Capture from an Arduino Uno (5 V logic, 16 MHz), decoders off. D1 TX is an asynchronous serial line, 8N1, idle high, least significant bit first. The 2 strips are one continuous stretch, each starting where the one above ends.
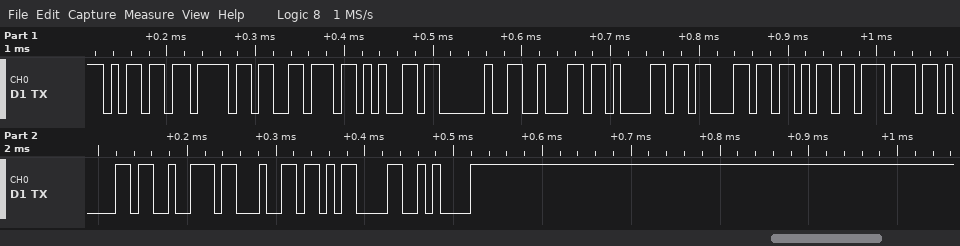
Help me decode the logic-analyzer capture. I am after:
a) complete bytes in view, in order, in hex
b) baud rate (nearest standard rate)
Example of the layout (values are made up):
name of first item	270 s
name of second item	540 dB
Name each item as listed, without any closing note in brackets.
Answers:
complete bytes in view, in order, in hex	0x6D 0x6F 0x76 0x65 0x20 0x62 0x61 0x63 0x6B 0x77 0x61 0x72 0x64 0x0D 0x0A
baud rate	115200 baud
